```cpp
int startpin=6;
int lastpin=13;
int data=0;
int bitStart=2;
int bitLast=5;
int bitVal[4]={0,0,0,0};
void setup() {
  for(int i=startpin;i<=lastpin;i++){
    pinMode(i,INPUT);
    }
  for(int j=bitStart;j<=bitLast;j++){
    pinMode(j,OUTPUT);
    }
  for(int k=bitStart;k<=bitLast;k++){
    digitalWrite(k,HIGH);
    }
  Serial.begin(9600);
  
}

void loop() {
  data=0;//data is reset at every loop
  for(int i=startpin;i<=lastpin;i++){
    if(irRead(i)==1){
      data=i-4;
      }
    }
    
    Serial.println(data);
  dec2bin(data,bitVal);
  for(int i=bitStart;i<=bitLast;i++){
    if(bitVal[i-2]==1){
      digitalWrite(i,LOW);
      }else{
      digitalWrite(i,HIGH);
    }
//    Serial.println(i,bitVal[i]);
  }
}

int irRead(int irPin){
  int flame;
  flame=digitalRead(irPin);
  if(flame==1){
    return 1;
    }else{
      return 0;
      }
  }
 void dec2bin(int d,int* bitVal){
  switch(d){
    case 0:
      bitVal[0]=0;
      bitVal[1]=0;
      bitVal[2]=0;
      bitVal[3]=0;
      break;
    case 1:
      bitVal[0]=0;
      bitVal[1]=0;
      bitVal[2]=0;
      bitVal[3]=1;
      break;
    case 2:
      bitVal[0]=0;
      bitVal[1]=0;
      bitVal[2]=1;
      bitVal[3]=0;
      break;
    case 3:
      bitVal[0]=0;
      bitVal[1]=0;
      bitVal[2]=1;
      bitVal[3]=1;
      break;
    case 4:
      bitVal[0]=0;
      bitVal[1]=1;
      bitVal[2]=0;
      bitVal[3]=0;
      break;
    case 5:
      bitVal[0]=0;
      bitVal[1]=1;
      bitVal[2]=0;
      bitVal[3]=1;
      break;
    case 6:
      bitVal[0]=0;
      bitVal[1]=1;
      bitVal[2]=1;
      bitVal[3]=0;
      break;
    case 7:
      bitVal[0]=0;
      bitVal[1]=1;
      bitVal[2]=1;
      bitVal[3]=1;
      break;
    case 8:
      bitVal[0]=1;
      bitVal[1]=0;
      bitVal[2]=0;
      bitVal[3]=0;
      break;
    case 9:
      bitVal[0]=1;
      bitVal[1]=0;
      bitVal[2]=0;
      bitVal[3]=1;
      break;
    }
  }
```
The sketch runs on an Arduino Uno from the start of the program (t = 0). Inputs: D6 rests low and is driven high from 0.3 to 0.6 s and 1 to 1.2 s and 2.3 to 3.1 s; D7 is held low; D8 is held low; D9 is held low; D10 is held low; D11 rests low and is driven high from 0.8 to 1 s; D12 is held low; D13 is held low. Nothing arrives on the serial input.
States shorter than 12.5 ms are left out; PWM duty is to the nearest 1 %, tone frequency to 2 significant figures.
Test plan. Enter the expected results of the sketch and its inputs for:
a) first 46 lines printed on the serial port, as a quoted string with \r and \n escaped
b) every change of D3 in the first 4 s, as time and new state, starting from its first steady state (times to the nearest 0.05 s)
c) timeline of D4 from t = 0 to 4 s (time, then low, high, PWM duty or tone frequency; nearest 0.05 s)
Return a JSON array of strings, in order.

["\"0\\r\\n0\\r\\n0\\r\\n0\\r\\n0\\r\\n0\\r\\n0\\r\\n0\\r\\n0\\r\\n0\\r\\n0\\r\\n0\\r\\n0\\r\\n0\\r\\n0\\r\\n0\\r\\n0\\r\\n0\\r\\n0\\r\\n0\\r\\n0\\r\\n0\\r\\n0\\r\\n0\\r\\n0\\r\\n0\\r\\n0\\r\\n0\\r\\n0\\r\\n0\\r\\n0\\r\\n0\\r\\n0\\r\\n0\\r\\n0\\r\\n0\\r\\n0\\r\\n0\\r\\n0\\r\\n0\\r\\n0\\r\\n0\\r\\n0\\r\\n0\\r\\n0\\r\\n0\\r\\n\"", "0 s high; 0.8 s low; 1 s high", "0 s high; 0.3 s low; 0.6 s high; 0.8 s low; 1.2 s high; 2.3 s low; 3.1 s high"]
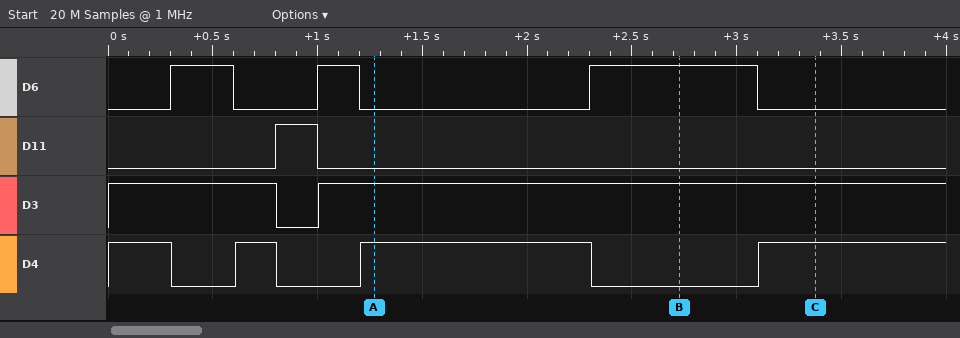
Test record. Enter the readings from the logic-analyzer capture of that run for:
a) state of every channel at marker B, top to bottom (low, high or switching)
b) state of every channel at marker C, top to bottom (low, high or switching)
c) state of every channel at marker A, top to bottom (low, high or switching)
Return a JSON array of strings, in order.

["D6 high, D11 low, D3 high, D4 low", "D6 low, D11 low, D3 high, D4 high", "D6 low, D11 low, D3 high, D4 high"]
